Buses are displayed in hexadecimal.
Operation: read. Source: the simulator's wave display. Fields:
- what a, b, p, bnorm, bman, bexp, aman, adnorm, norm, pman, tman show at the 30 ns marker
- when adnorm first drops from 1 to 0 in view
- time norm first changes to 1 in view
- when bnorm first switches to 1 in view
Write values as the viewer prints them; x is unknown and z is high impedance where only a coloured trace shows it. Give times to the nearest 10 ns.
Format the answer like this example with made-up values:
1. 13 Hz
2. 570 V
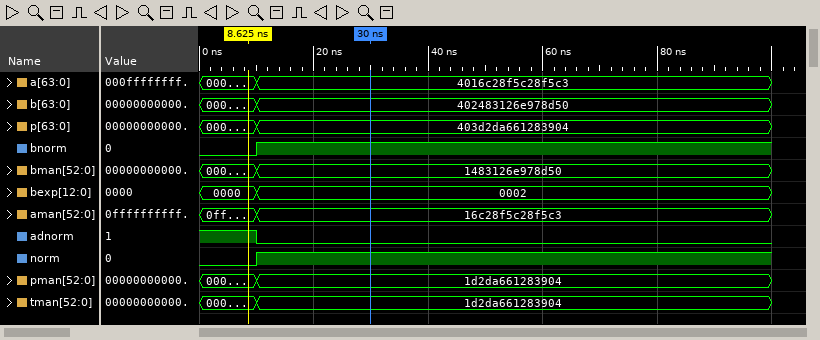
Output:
1. a=4016c28f5c28f5c3, b=402483126e978d50, p=403d2da661283904, bnorm=1, bman=1483126e978d50, bexp=0002, aman=16c28f5c28f5c3, adnorm=0, norm=1, pman=1d2da661283904, tman=1d2da661283904
2. 10 ns
3. 10 ns
4. 10 ns
